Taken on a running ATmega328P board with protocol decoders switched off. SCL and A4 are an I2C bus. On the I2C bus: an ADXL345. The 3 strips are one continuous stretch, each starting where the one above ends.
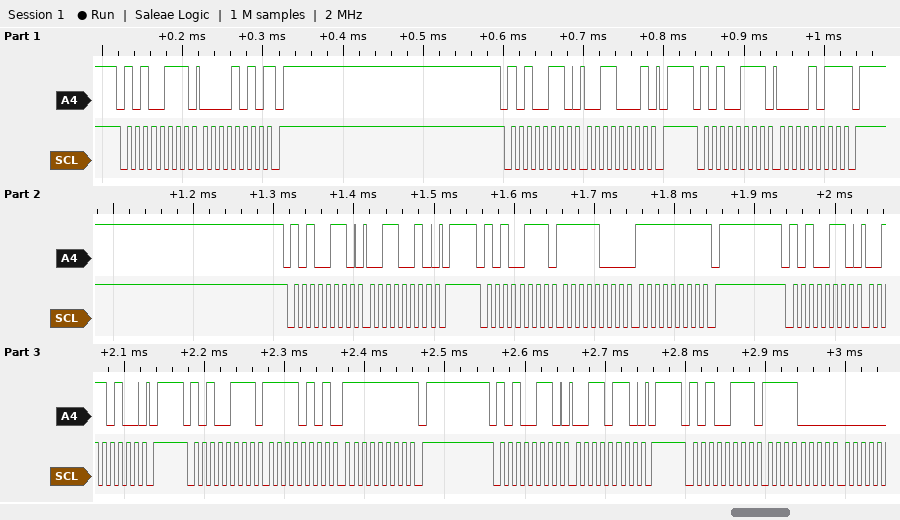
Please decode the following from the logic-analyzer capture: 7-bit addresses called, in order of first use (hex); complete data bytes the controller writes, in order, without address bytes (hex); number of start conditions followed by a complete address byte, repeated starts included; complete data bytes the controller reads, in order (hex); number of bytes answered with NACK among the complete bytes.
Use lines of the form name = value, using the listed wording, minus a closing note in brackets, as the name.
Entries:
7-bit addresses called, in order of first use = 0x53
complete data bytes the controller writes, in order, without address bytes = 31 32 34 36
number of start conditions followed by a complete address byte, repeated starts included = 9
complete data bytes the controller reads, in order = 0A 0B F8 FF F5 FF F0
number of bytes answered with NACK among the complete bytes = 4
